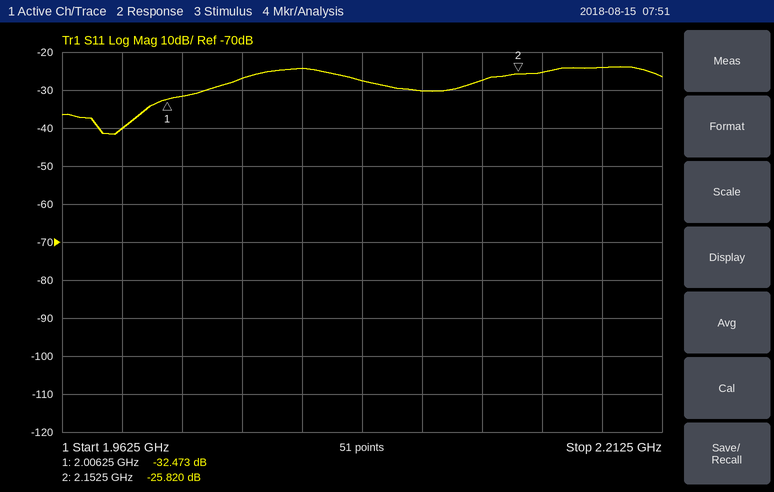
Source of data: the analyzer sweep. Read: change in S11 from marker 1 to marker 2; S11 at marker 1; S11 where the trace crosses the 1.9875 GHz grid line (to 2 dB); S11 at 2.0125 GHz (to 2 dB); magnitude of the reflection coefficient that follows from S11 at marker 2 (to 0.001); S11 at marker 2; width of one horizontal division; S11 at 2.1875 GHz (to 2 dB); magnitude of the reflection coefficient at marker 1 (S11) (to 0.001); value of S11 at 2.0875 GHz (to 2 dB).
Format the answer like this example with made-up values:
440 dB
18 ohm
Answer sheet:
6.653 dB
-32.473 dB
-40 dB
-32 dB
0.051
-25.820 dB
25 MHz
-24 dB
0.024
-28 dB
